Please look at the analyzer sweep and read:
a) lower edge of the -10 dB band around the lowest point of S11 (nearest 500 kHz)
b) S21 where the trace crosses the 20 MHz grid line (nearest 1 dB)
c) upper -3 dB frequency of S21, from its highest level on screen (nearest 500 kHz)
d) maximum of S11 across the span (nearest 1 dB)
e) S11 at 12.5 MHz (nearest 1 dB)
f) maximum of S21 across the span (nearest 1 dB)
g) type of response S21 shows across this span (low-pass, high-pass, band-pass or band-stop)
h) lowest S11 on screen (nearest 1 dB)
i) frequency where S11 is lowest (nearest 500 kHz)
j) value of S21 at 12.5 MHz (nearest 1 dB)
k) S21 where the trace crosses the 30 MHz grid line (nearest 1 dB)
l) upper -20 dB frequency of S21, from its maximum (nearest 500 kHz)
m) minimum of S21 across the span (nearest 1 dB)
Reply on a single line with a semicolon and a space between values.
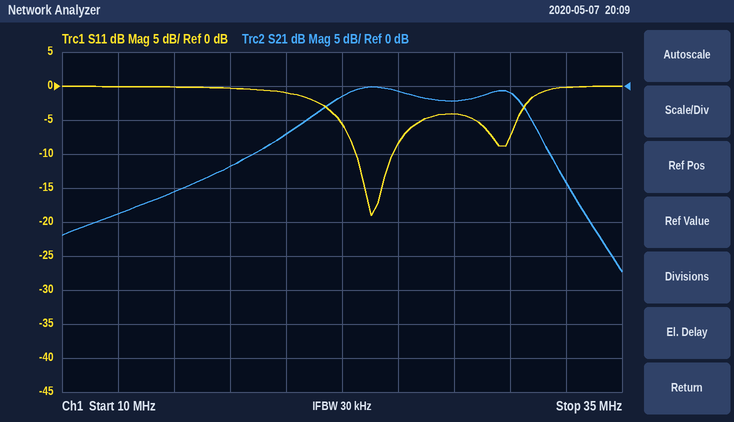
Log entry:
23.0 MHz; -7 dB; 30.5 MHz; 0 dB; 0 dB; 0 dB; band-pass; -19 dB; 24.0 MHz; -19 dB; -1 dB; 33.5 MHz; -27 dB
